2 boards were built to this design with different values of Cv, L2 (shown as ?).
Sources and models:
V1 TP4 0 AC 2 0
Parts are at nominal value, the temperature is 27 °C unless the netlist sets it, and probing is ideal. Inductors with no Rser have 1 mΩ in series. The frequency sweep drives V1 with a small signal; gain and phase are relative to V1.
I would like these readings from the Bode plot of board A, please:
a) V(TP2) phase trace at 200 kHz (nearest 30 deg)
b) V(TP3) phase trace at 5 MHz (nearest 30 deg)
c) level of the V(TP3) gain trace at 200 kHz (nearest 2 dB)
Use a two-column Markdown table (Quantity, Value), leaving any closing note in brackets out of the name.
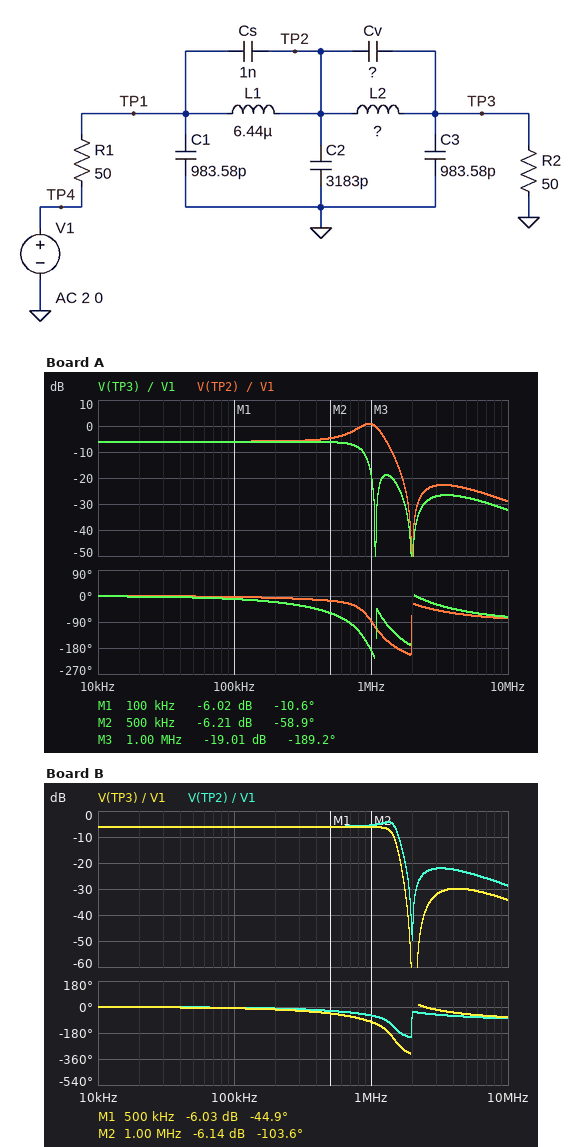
| Quantity | Value |
|---|---|
| V(TP2) phase trace at 200 kHz | 0 deg |
| V(TP3) phase trace at 5 MHz | -60 deg |
| level of the V(TP3) gain trace at 200 kHz | -6 dB |
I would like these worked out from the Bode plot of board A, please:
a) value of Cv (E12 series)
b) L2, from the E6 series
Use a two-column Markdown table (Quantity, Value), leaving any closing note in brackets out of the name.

| Quantity | Value |
|---|---|
| value of Cv | 2.2 nF |
| L2, from the E6 series | 10 µH |
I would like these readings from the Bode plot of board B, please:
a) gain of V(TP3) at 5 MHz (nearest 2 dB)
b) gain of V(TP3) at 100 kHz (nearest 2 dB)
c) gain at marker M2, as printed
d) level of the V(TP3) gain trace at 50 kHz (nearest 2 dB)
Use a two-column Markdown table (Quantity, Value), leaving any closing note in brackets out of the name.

| Quantity | Value |
|---|---|
| gain of V(TP3) at 5 MHz | -30 dB |
| gain of V(TP3) at 100 kHz | -6 dB |
| gain at marker M2, as printed | -6.14 dB |
| level of the V(TP3) gain trace at 50 kHz | -6 dB |
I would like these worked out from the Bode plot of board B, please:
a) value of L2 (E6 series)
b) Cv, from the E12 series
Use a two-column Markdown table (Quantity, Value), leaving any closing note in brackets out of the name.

| Quantity | Value |
|---|---|
| value of L2 | 4.7 µH |
| Cv, from the E12 series | 1.2 nF |
